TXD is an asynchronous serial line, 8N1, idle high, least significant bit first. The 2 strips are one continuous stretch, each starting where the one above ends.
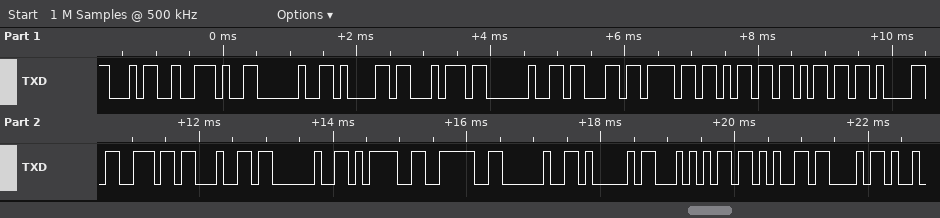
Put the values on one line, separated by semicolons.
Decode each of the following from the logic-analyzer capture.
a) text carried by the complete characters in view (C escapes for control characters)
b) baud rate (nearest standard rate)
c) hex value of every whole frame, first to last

"4. at command => AT+C"; 9600 baud; 34 2E 20 61 74 20 63 6F 6D 6D 61 6E 64 20 3D 3E 20 41 54 2B 43
